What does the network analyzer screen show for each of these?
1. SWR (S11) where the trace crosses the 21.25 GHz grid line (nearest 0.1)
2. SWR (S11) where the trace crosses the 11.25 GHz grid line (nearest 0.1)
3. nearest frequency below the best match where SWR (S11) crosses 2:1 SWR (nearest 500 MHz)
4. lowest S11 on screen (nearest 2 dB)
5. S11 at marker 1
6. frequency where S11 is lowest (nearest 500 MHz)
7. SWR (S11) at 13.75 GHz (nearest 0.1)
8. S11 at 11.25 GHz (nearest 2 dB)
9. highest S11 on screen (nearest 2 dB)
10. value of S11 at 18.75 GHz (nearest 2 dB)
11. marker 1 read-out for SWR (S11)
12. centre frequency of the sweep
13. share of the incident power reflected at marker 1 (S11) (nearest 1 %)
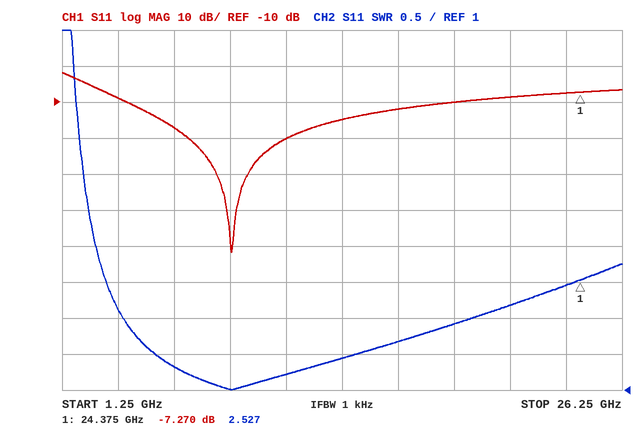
2.2
1.2
4.0 GHz
-52 dB
-7.270 dB
9.0 GHz
1.4
-20 dB
-2 dB
-10 dB
2.527
13.75 GHz
19 %
